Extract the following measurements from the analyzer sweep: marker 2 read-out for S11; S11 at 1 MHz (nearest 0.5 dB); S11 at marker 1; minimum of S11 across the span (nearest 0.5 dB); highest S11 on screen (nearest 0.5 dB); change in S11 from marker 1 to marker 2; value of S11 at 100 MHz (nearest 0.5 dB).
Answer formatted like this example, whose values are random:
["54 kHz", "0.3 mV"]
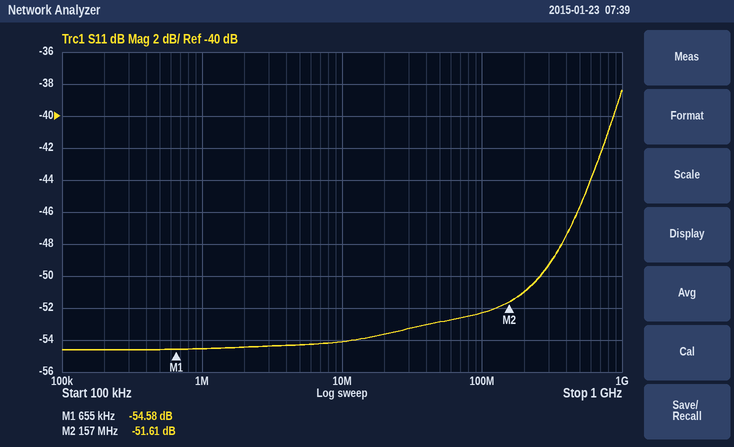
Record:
["-51.61 dB", "-54.5 dB", "-54.58 dB", "-54.5 dB", "-38.5 dB", "2.97 dB", "-52.5 dB"]
